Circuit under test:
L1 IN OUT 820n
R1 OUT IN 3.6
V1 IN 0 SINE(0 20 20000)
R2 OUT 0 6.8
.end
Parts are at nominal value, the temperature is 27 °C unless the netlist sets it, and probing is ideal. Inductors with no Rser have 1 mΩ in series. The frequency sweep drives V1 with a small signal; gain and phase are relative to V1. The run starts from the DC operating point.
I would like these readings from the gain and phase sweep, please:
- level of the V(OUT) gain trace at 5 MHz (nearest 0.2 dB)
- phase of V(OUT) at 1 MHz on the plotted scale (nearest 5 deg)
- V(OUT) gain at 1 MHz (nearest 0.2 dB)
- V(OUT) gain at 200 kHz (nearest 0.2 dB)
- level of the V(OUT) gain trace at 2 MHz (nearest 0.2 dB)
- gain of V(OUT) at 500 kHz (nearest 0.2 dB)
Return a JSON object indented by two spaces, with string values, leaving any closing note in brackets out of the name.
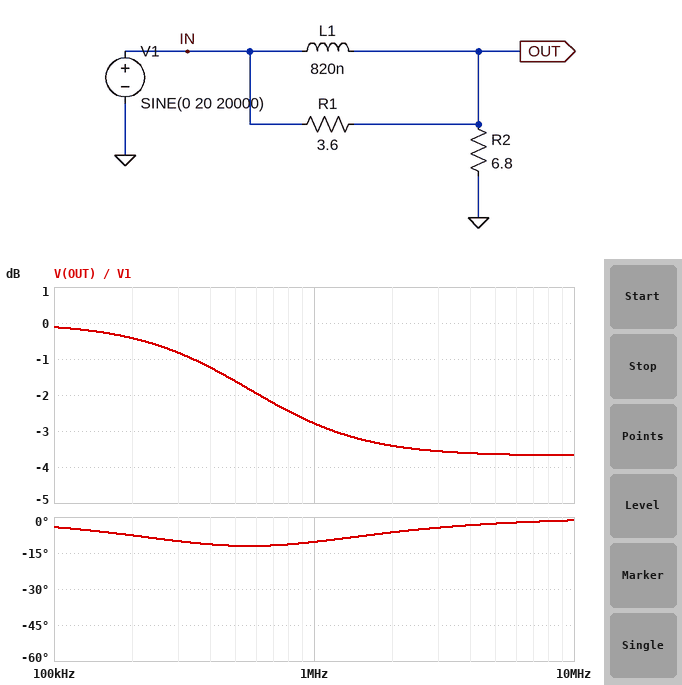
{
  "level of the V(OUT) gain trace at 5 MHz": "-3.6 dB",
  "phase of V(OUT) at 1 MHz on the plotted scale": "-10 deg",
  "V(OUT) gain at 1 MHz": "-2.8 dB",
  "V(OUT) gain at 200 kHz": "-0.4 dB",
  "level of the V(OUT) gain trace at 2 MHz": "-3.4 dB",
  "gain of V(OUT) at 500 kHz": "-1.6 dB"
}
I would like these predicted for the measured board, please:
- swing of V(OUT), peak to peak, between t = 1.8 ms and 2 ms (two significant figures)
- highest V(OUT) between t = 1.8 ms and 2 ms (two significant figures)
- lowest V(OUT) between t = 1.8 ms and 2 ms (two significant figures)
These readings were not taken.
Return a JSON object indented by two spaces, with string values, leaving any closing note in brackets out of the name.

{
  "swing of V(OUT), peak to peak, between t = 1.8 ms and 2 ms": "40 V",
  "highest V(OUT) between t = 1.8 ms and 2 ms": "20 V",
  "lowest V(OUT) between t = 1.8 ms and 2 ms": "-20 V"
}
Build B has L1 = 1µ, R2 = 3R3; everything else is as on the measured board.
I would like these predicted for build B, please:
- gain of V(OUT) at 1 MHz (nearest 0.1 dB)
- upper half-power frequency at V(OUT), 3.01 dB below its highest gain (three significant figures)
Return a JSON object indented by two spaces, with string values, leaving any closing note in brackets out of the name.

{
  "gain of V(OUT) at 1 MHz": "-5.5 dB",
  "upper half-power frequency at V(OUT), 3.01 dB below its highest gain": "372 kHz"
}
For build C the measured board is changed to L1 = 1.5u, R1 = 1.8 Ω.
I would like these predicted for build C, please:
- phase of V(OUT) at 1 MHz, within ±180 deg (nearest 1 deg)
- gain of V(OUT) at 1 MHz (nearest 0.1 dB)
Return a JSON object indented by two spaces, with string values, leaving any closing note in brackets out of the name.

{
  "phase of V(OUT) at 1 MHz, within ±180 deg": "-2 deg",
  "gain of V(OUT) at 1 MHz": "-2.0 dB"
}
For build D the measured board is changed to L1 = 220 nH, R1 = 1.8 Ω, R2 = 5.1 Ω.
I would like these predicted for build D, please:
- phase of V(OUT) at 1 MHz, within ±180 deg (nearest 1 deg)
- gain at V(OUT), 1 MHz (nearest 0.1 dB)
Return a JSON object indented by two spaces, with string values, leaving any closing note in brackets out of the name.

{
  "phase of V(OUT) at 1 MHz, within ±180 deg": "-9 deg",
  "gain at V(OUT), 1 MHz": "-1.2 dB"
}
